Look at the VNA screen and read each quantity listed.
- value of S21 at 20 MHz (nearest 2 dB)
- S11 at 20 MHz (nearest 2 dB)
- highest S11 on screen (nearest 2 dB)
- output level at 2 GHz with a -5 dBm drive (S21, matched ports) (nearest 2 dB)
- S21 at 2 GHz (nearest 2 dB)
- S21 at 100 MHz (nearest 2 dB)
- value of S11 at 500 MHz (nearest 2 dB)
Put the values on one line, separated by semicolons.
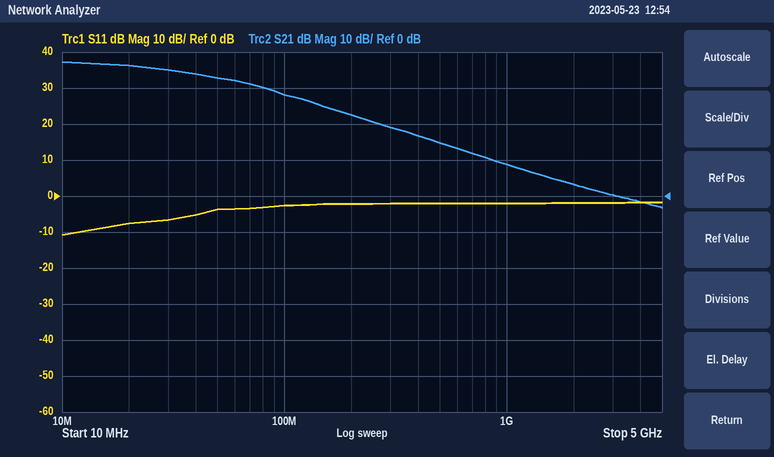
36 dB; -8 dB; -2 dB; -2 dBm; 4 dB; 28 dB; -2 dB
